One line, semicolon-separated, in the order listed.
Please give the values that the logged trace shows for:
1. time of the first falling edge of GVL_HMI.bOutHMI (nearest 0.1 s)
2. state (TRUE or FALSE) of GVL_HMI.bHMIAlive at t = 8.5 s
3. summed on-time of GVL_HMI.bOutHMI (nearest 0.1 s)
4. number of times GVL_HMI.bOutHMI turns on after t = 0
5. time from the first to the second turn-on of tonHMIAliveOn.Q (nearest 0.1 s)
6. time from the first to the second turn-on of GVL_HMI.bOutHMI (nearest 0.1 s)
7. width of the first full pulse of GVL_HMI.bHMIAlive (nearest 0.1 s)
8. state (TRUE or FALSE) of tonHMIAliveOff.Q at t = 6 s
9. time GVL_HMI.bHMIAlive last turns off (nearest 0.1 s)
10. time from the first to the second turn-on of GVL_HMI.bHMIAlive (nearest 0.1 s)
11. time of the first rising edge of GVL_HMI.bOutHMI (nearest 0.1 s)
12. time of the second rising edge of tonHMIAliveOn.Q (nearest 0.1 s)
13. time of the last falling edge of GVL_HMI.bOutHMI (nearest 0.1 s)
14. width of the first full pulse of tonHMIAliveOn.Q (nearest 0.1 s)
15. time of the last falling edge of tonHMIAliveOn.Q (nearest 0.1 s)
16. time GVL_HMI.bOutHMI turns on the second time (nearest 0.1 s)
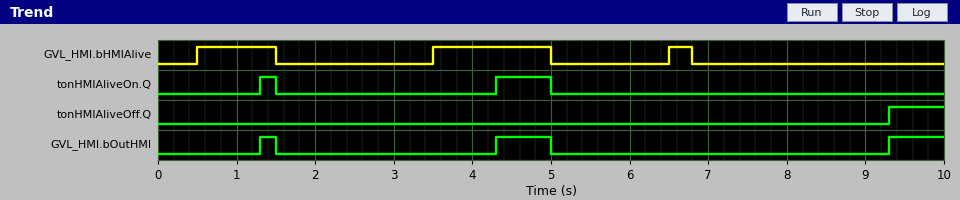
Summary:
1.5 s; FALSE; 1.6 s; 3; 3.0 s; 3.0 s; 1.0 s; FALSE; 6.8 s; 3.0 s; 1.3 s; 4.3 s; 5.0 s; 0.2 s; 5.0 s; 4.3 s
